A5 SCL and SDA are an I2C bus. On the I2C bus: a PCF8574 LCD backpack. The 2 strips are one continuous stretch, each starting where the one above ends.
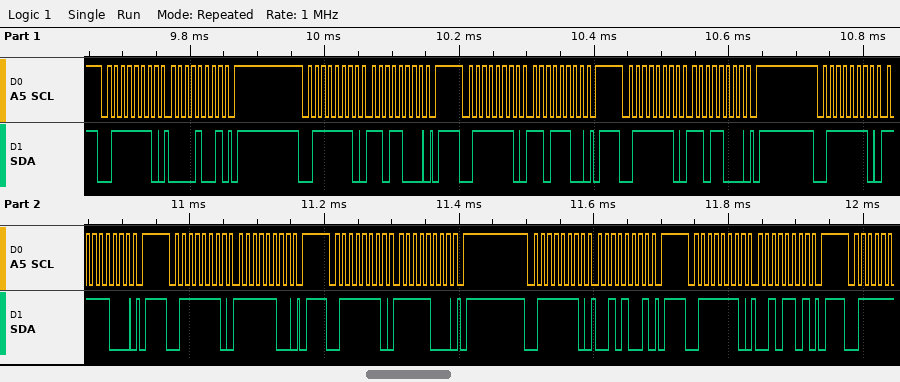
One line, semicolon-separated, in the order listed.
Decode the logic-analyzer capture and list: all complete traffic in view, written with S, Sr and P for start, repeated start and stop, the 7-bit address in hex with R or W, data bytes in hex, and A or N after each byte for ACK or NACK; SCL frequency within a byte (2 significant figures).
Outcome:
S 3FW A 09 A P S 3FW A D8 A P S 3FW A DC A P S 3FW A D8 A P S 3FW A F8 A P S 3FW A FC A P S 3FW A F8 A P S 3FW A 29 A P S 3FW A 2D A P; 100 kHz
